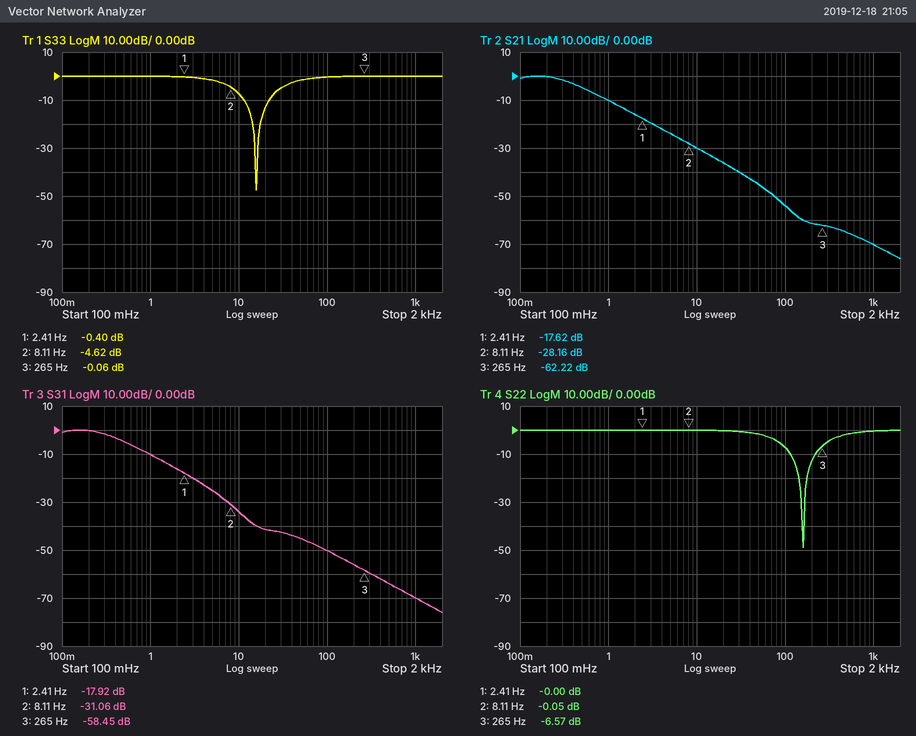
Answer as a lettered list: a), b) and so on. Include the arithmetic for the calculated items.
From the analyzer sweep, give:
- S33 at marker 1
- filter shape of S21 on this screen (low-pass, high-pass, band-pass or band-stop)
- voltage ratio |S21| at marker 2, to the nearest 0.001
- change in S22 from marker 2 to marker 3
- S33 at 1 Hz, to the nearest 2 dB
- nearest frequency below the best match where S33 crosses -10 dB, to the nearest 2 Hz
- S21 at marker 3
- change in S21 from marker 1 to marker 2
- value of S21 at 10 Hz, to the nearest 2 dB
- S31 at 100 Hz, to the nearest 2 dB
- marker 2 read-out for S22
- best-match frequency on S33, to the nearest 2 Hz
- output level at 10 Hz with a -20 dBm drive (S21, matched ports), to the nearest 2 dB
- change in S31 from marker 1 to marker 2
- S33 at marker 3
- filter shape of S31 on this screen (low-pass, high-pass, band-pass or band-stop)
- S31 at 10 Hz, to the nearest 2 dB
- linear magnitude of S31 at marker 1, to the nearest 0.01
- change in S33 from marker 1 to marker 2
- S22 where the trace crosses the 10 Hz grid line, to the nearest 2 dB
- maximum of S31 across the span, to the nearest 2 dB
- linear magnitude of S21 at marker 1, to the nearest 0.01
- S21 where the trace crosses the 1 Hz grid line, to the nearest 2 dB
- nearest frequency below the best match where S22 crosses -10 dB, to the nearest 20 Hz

a) -0.40 dB
b) low-pass
c) 10^(-28.16/20) ≈ 0.039
d) -6.57 − (-0.05) = -6.52 dB
e) 0 dB
f) 12 Hz
g) -62.22 dB
h) -28.16 − (-17.62) = -10.54 dB
i) -30 dB
j) -50 dB
k) -0.05 dB
l) 16 Hz
m) -20 dBm + (-30 dB) = -50 dBm
n) -31.06 − (-17.92) = -13.14 dB
o) -0.06 dB
p) low-pass
q) -34 dB
r) 10^(-17.92/20) ≈ 0.13
s) -4.62 − (-0.4) = -4.22 dB
t) 0 dB
u) 0 dB
v) 10^(-17.62/20) ≈ 0.13
w) -10 dB
x) 120 Hz
